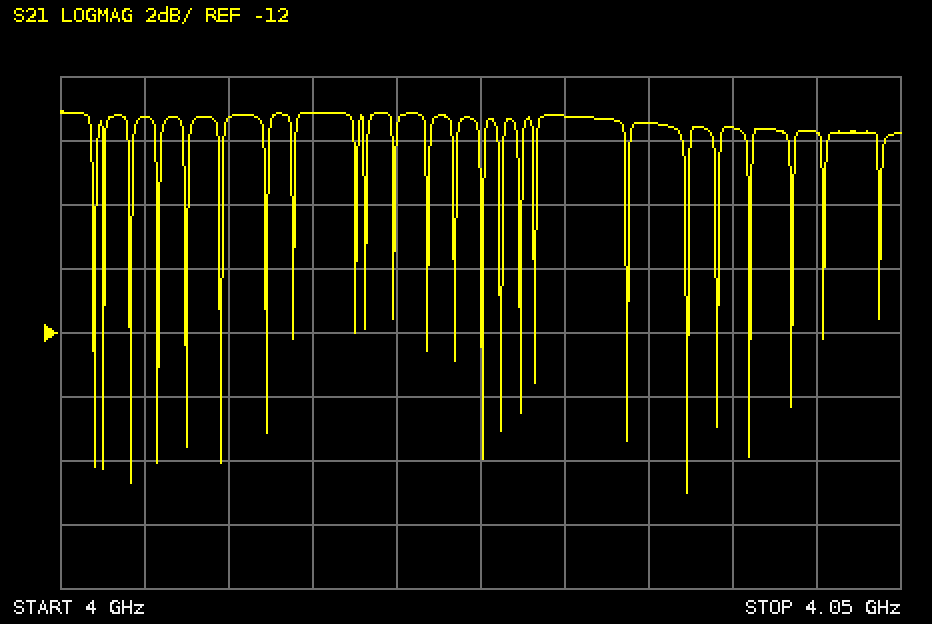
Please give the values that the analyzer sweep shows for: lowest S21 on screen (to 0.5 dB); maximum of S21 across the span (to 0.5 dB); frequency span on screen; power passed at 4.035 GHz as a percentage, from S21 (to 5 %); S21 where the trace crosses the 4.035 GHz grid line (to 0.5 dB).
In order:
-17.0 dB
-5.0 dB
50 MHz
30 %
-5.5 dB
